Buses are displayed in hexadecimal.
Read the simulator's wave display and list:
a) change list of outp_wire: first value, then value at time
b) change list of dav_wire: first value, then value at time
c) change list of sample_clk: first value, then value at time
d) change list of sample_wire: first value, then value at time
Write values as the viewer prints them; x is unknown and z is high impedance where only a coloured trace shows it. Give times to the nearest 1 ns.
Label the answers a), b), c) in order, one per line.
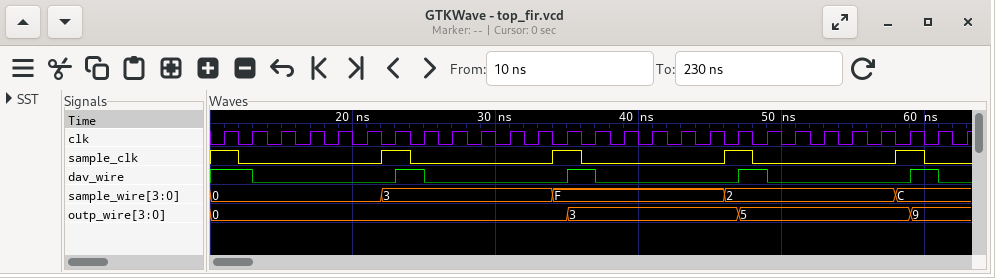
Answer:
a) 0, 3 at 35 ns, 5 at 47 ns, 9 at 59 ns
b) 1, 0 at 13 ns, 1 at 23 ns, 0 at 25 ns, 1 at 35 ns, 0 at 37 ns, 1 at 47 ns, 0 at 49 ns, 1 at 59 ns, 0 at 61 ns
c) 1, 0 at 12 ns, 1 at 22 ns, 0 at 24 ns, 1 at 34 ns, 0 at 36 ns, 1 at 46 ns, 0 at 48 ns, 1 at 58 ns, 0 at 60 ns
d) 0, 3 at 22 ns, F at 34 ns, 2 at 46 ns, C at 58 ns
